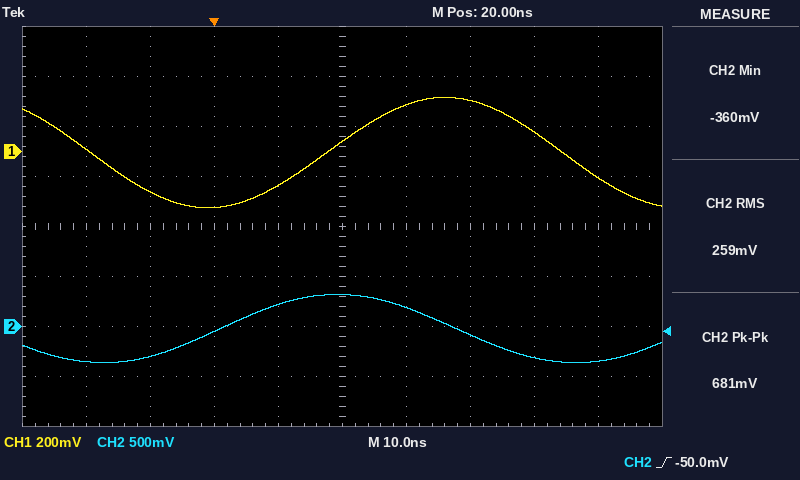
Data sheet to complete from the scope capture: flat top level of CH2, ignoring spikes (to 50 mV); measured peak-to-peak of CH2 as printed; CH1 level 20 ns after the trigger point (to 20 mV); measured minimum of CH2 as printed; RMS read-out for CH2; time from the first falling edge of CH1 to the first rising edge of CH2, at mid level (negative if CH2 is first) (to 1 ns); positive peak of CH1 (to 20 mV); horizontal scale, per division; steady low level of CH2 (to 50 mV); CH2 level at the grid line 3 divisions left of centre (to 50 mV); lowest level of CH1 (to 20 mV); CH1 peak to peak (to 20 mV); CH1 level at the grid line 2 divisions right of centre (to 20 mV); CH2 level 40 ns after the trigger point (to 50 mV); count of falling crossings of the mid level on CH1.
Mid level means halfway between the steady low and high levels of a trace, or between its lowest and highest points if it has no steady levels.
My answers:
300 mV
681 mV
40 mV
-360 mV
259 mV
+20 ns
220 mV
10 ns
-350 mV
-300 mV
-220 mV
440 mV
200 mV
-100 mV
2
